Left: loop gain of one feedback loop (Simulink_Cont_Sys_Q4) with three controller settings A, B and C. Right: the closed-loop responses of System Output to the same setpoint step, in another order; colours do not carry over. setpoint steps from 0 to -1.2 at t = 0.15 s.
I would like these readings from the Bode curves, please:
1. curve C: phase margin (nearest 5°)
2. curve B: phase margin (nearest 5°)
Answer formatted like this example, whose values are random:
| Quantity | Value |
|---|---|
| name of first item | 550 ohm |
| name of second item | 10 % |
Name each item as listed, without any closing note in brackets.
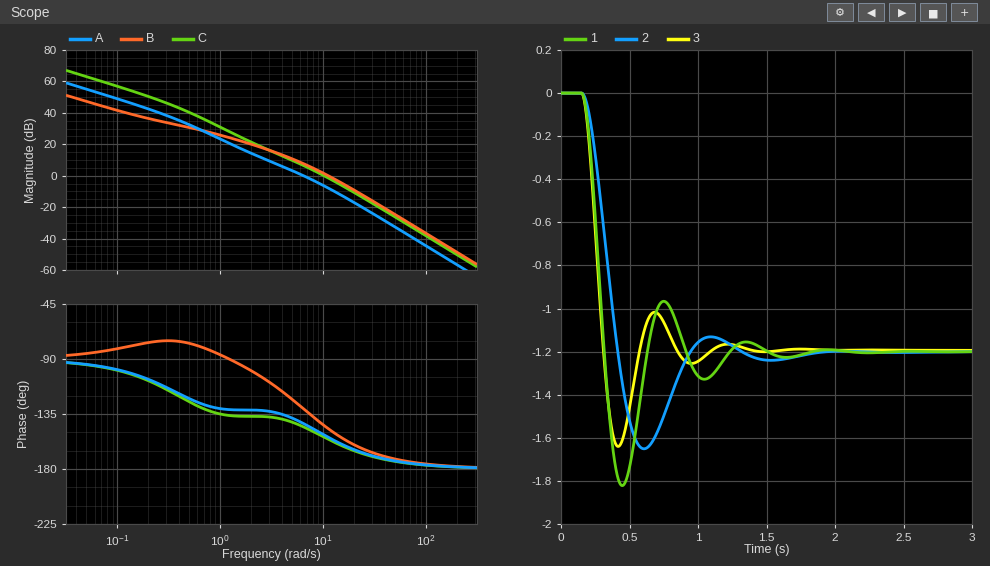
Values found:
| Quantity | Value |
|---|---|
| curve C: phase margin | 25° |
| curve B: phase margin | 35° |
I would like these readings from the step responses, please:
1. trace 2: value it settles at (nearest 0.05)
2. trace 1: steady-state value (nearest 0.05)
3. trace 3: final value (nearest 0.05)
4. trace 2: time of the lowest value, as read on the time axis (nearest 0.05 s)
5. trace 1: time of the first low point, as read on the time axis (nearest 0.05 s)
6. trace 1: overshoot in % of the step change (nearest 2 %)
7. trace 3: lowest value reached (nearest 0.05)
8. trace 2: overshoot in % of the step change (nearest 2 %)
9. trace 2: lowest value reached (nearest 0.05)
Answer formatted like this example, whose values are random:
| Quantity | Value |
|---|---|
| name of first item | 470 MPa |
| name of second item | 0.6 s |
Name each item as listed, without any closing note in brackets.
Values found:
| Quantity | Value |
|---|---|
| trace 2: value it settles at | -1.20 |
| trace 1: steady-state value | -1.20 |
| trace 3: final value | -1.20 |
| trace 2: time of the lowest value, as read on the time axis | 0.60 s |
| trace 1: time of the first low point, as read on the time axis | 0.45 s |
| trace 1: overshoot in % of the step change | 52 % |
| trace 3: lowest value reached | -1.65 |
| trace 2: overshoot in % of the step change | 38 % |
| trace 2: lowest value reached | -1.65 |
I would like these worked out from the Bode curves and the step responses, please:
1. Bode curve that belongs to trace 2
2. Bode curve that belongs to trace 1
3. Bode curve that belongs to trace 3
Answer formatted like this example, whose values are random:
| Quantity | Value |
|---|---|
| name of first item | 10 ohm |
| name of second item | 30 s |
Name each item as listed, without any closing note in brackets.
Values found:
| Quantity | Value |
|---|---|
| Bode curve that belongs to trace 2 | A |
| Bode curve that belongs to trace 1 | C |
| Bode curve that belongs to trace 3 | B |
